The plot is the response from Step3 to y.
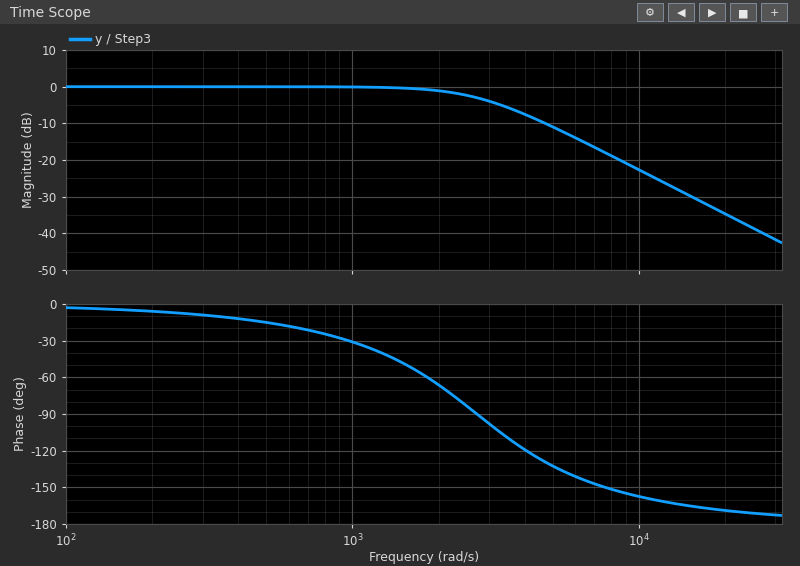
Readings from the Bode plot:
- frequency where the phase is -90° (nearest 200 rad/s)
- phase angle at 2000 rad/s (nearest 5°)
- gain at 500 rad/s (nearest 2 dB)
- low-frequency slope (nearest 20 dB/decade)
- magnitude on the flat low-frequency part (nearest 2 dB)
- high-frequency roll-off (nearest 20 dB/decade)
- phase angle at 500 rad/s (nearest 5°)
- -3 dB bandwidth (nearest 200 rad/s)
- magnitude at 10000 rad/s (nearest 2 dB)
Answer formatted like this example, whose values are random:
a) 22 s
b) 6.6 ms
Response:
a) 2800 rad/s
b) -65°
c) 0 dB
d) 0 dB/decade
e) 0 dB
f) -40 dB/decade
g) -15°
h) 2800 rad/s
i) -22 dB
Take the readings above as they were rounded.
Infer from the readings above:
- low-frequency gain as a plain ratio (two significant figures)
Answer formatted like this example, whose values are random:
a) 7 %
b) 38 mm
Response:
a) 1.0
